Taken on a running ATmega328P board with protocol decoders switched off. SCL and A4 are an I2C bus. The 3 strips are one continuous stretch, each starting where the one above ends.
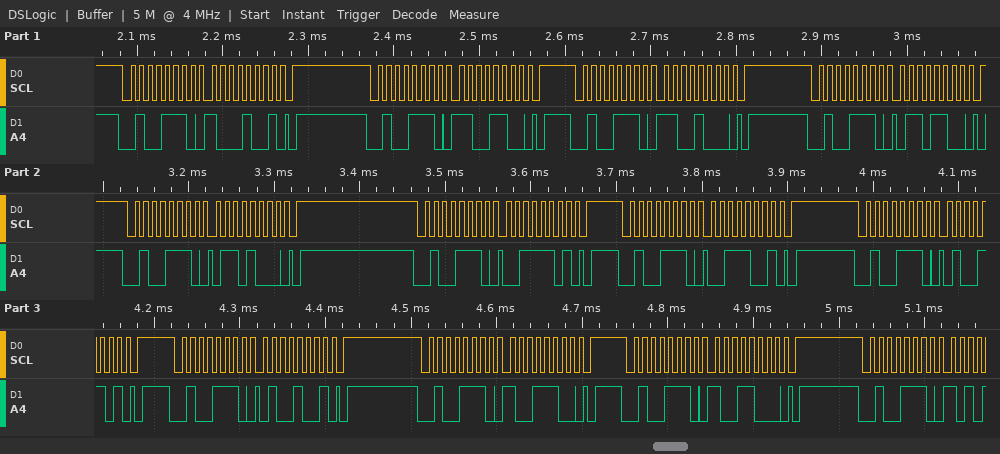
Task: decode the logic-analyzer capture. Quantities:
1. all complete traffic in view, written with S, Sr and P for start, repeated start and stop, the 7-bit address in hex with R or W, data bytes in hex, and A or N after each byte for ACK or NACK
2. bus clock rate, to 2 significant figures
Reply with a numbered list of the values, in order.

1. S 27W A 89 A P S 27W A CC A P S 27W A C8 A P S 27W A 6C A P S 27W A 68 A P S 27W A 3D A P S 27W A 39 A P S 27W A 4D A P S 27W A 49 A P S 27W A 9C A P S 27W A 98 A P S 27W A
2. 100 kHz
